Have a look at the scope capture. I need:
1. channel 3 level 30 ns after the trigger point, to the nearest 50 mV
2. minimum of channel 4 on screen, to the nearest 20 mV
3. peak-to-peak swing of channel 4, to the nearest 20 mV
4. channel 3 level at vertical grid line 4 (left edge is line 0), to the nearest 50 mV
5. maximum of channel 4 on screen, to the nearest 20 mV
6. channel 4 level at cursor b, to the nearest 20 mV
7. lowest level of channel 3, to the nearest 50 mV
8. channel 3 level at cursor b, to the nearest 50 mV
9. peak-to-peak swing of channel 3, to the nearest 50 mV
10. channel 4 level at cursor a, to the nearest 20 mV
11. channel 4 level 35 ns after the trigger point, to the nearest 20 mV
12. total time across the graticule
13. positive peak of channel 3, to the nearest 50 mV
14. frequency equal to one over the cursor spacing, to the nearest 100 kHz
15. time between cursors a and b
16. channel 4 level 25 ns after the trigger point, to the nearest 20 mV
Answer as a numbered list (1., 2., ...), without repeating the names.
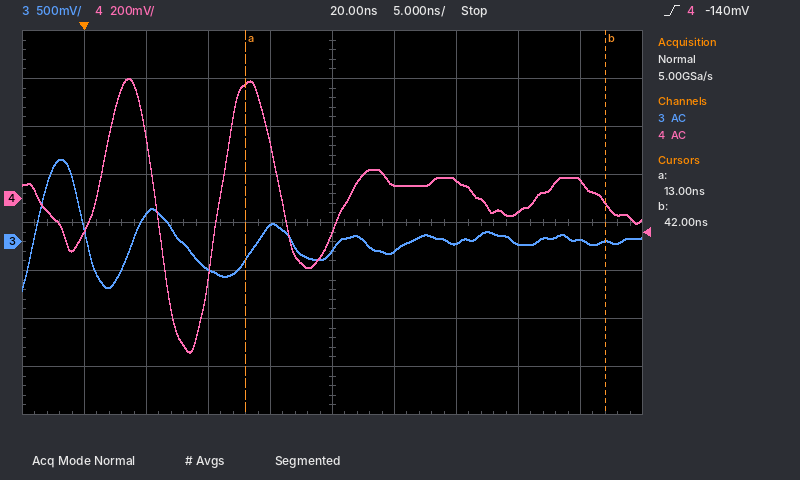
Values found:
1. 0 mV
2. -640 mV
3. 1.14 V
4. 150 mV
5. 500 mV
6. -20 mV
7. -500 mV
8. 0 mV
9. 1.35 V
10. 480 mV
11. -60 mV
12. 50 ns
13. 850 mV
14. 34.5 MHz
15. 29.0 ns
16. 60 mV
